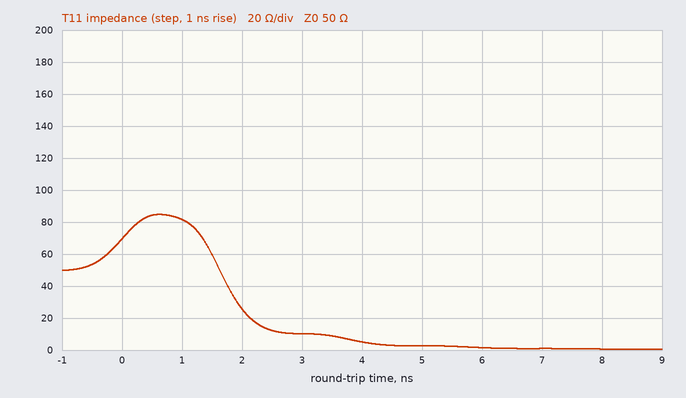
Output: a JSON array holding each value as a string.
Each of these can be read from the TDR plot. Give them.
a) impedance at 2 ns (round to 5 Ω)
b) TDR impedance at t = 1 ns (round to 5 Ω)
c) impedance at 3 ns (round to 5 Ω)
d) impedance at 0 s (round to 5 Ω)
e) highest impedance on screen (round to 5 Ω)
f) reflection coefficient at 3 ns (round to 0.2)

["25 Ω", "80 Ω", "10 Ω", "70 Ω", "85 Ω", "-0.6"]
